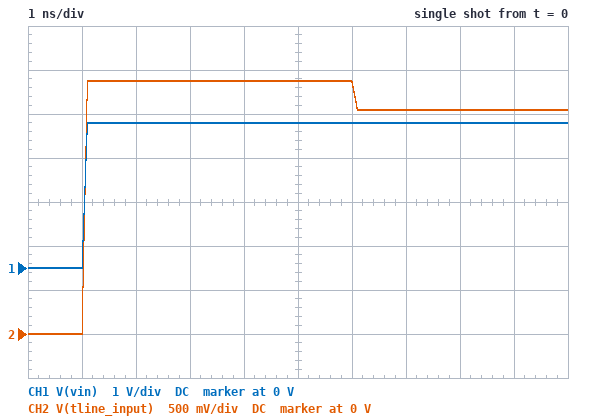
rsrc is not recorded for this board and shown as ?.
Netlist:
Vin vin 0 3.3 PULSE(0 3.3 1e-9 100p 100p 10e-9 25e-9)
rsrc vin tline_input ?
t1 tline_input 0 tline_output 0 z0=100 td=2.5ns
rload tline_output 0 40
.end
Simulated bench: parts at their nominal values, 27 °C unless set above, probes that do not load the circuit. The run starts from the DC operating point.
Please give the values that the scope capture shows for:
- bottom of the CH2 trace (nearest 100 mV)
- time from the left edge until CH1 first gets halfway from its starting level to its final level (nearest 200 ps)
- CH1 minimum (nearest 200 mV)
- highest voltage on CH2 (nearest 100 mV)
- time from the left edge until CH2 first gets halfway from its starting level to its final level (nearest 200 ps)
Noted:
0 V
1.0 ns
0 V
2.9 V
1.0 ns
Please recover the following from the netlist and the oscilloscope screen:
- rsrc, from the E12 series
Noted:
15 Ω
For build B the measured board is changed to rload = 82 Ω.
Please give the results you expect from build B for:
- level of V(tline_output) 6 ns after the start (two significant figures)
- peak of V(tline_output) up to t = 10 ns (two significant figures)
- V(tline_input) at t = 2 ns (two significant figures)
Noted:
2.6 V
2.8 V
2.9 V
